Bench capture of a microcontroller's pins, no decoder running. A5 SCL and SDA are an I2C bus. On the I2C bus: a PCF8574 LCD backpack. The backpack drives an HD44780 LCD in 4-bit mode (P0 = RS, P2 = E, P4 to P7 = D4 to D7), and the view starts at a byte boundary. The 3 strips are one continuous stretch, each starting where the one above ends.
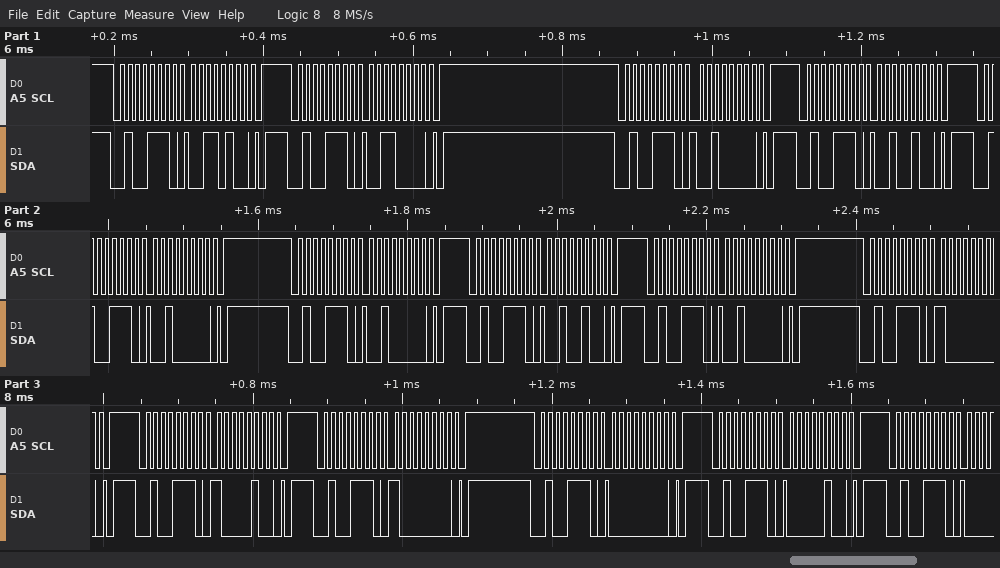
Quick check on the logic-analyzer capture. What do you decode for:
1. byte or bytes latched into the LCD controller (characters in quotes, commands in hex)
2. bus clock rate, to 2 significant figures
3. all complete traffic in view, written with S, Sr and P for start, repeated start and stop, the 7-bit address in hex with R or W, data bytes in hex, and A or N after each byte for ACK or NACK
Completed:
0x28
100 kHz
S 27W A 34 A P S 27W A 30 A P S 27W A 20 A P S 27W A 24 A P S 27W A 20 A P S 27W A 20 A P S 27W A 24 A P S 27W A 20 A P S 27W A 80 A P S 27W A 84 A P S 27W A 80 A P S 27W A 00 A P S 27W A 04 A P S 27W A
